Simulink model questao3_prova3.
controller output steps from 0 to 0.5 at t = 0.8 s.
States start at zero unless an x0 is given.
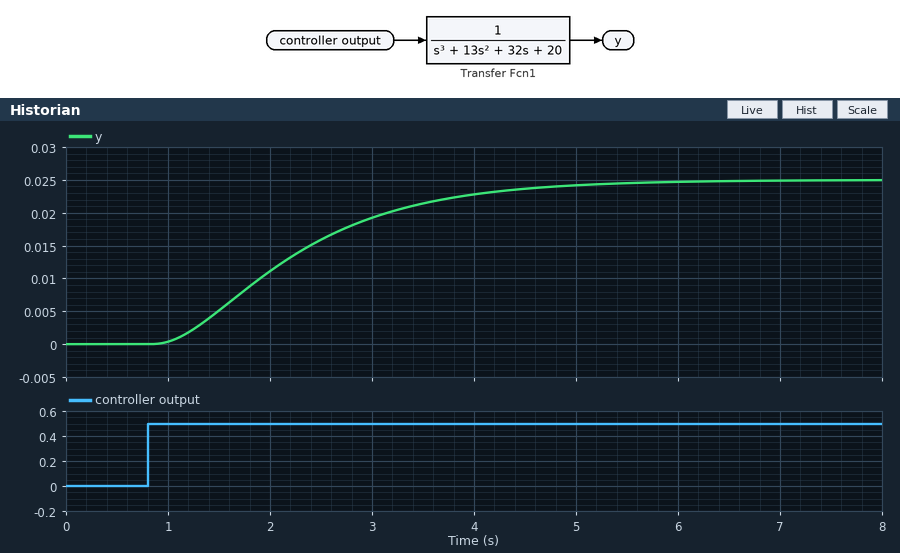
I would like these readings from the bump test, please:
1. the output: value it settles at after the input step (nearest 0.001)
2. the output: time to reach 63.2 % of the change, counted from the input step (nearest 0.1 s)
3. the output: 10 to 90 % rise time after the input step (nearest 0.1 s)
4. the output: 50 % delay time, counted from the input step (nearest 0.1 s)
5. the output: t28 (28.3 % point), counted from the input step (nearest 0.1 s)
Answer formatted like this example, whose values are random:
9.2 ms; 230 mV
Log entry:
0.025; 1.7 s; 2.6 s; 1.3 s; 0.9 s
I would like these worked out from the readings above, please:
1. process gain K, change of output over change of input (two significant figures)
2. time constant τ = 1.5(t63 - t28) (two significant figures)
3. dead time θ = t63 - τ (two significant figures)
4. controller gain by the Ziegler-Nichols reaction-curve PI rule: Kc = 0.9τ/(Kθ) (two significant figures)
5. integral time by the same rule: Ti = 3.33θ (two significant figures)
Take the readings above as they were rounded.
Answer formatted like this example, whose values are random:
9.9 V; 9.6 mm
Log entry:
0.050; 1.2 s; 0.50 s; 43; 1.7 s
